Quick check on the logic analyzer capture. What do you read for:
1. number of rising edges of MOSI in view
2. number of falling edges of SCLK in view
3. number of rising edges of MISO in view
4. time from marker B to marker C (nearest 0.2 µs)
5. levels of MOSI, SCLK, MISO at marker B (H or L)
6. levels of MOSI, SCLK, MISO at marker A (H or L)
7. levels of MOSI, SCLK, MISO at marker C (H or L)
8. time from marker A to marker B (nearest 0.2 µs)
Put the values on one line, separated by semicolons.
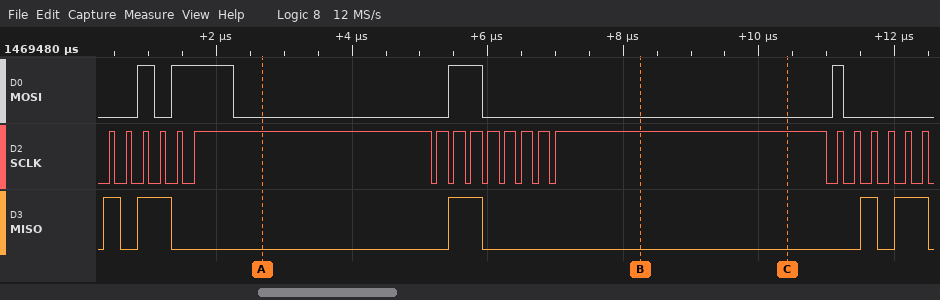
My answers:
4; 20; 5; 2.2 µs; MOSI=L, SCLK=H, MISO=L; MOSI=L, SCLK=H, MISO=L; MOSI=L, SCLK=H, MISO=L; 5.6 µs
